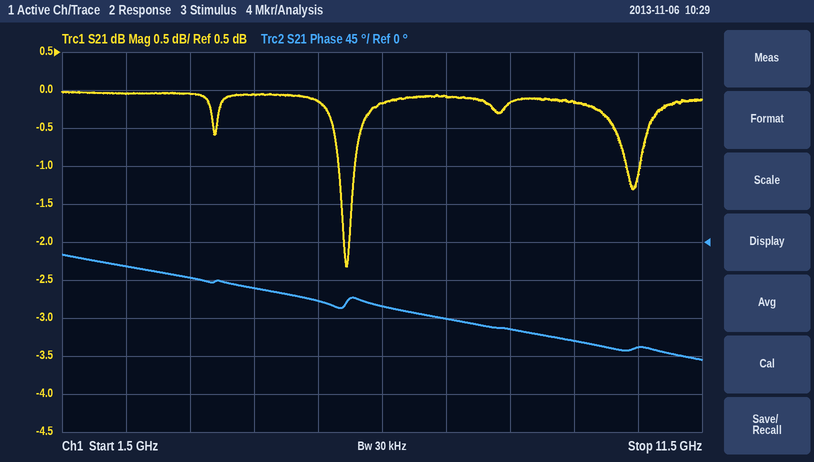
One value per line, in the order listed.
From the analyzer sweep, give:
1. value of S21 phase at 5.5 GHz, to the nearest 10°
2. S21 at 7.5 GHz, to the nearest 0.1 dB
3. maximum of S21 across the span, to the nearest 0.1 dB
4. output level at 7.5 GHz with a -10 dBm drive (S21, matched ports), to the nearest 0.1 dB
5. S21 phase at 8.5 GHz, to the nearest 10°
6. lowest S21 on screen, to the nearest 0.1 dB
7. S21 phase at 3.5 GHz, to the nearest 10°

-70°
-0.1 dB
0.0 dB
-10.1 dBm
-100°
-2.3 dB
-40°
